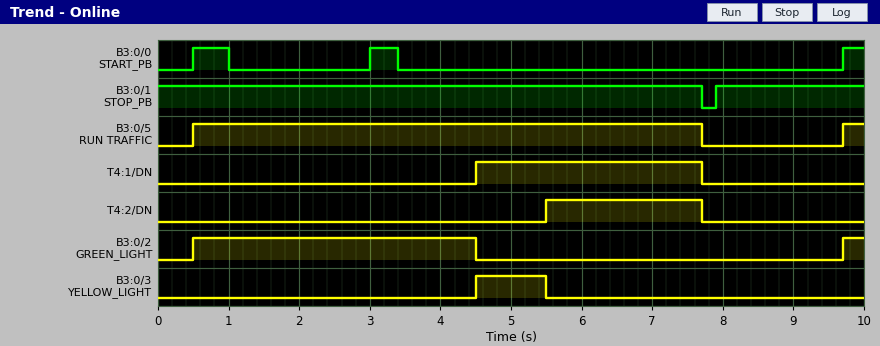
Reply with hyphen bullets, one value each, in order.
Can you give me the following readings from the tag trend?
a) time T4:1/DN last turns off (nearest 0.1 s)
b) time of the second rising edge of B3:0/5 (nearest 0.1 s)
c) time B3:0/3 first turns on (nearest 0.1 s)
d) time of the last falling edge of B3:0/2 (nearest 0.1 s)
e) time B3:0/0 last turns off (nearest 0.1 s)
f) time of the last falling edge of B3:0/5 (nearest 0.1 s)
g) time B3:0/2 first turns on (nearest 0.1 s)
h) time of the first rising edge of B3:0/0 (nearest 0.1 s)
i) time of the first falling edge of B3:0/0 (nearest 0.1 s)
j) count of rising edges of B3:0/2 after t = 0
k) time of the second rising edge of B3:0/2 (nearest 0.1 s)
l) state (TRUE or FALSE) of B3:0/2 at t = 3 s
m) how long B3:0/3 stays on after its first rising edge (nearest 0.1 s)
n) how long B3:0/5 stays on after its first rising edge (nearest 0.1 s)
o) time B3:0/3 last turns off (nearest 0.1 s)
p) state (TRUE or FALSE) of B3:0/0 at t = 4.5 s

- 7.7 s
- 9.7 s
- 4.5 s
- 4.5 s
- 3.4 s
- 7.7 s
- 0.5 s
- 0.5 s
- 1.0 s
- 2
- 9.7 s
- TRUE
- 1.0 s
- 7.2 s
- 5.5 s
- FALSE
